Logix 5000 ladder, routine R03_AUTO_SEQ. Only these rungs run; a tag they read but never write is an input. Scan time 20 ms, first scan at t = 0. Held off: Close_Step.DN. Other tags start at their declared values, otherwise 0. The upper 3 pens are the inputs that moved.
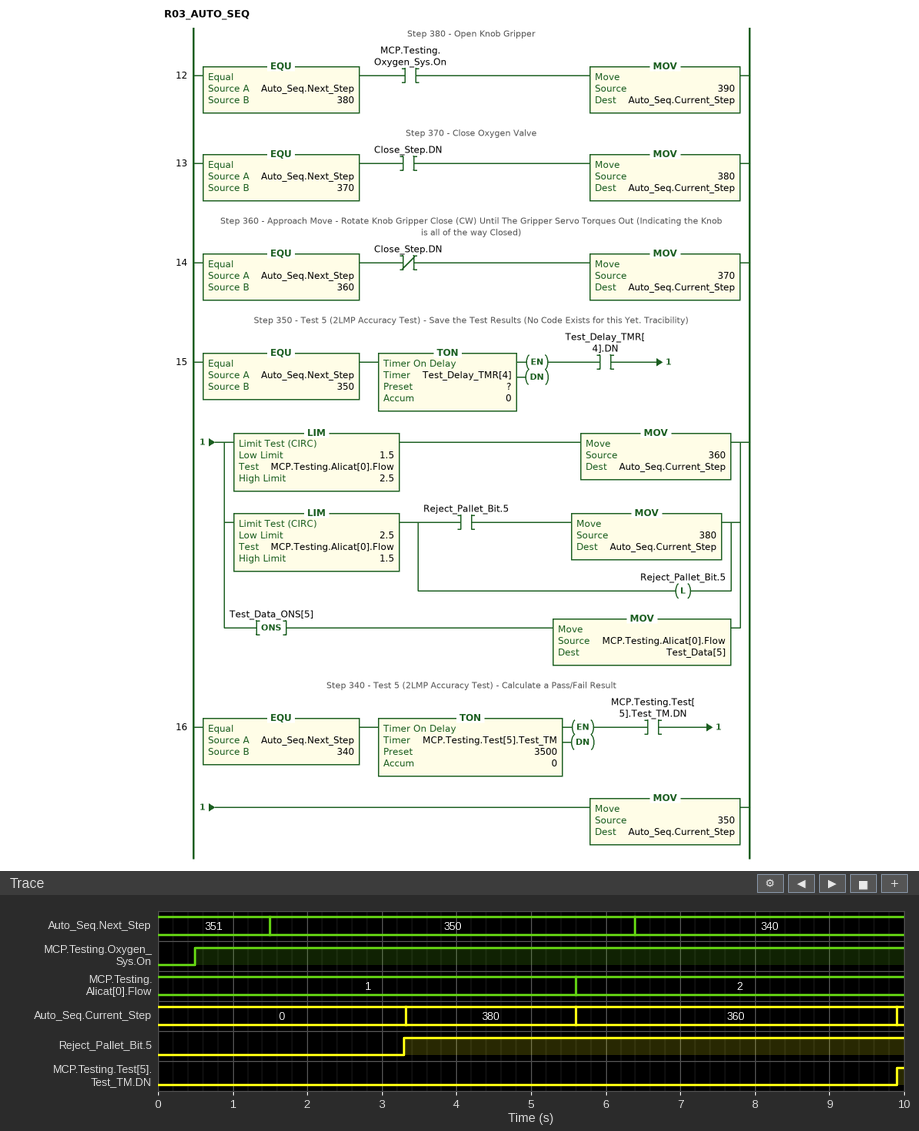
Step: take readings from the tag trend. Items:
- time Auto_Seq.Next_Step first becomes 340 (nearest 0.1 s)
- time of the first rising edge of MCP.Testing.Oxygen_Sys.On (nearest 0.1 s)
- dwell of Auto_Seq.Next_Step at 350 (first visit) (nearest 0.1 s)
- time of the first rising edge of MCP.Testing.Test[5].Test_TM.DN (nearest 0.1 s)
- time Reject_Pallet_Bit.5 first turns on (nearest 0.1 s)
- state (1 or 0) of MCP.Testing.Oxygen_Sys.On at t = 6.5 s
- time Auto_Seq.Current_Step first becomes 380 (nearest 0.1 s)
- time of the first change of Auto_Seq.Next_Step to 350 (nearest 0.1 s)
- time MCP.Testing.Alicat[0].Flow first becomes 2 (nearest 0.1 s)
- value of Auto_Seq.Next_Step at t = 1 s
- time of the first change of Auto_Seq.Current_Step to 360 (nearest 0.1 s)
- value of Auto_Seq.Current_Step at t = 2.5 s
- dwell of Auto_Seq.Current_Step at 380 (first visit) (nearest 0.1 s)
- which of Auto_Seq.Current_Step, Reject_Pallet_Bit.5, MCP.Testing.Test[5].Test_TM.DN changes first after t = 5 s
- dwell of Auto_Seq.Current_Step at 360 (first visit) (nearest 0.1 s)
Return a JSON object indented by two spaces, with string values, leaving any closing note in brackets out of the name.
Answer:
{
  "time Auto_Seq.Next_Step first becomes 340": "6.4 s",
  "time of the first rising edge of MCP.Testing.Oxygen_Sys.On": "0.5 s",
  "dwell of Auto_Seq.Next_Step at 350 (first visit)": "4.9 s",
  "time of the first rising edge of MCP.Testing.Test[5].Test_TM.DN": "9.9 s",
  "time Reject_Pallet_Bit.5 first turns on": "3.3 s",
  "state (1 or 0) of MCP.Testing.Oxygen_Sys.On at t = 6.5 s": "1",
  "time Auto_Seq.Current_Step first becomes 380": "3.3 s",
  "time of the first change of Auto_Seq.Next_Step to 350": "1.5 s",
  "time MCP.Testing.Alicat[0].Flow first becomes 2": "5.6 s",
  "value of Auto_Seq.Next_Step at t = 1 s": "351",
  "time of the first change of Auto_Seq.Current_Step to 360": "5.6 s",
  "value of Auto_Seq.Current_Step at t = 2.5 s": "0",
  "dwell of Auto_Seq.Current_Step at 380 (first visit)": "2.3 s",
  "which of Auto_Seq.Current_Step, Reject_Pallet_Bit.5, MCP.Testing.Test[5].Test_TM.DN changes first after t = 5 s": "Auto_Seq.Current_Step",
  "dwell of Auto_Seq.Current_Step at 360 (first visit)": "4.3 s"
}
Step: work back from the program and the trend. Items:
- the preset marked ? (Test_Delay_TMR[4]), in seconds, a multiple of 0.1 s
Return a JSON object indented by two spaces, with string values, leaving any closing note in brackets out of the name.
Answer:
{
  "the preset marked ? (Test_Delay_TMR[4]), in seconds, a multiple of 0.1 s": "1.8 s"
}
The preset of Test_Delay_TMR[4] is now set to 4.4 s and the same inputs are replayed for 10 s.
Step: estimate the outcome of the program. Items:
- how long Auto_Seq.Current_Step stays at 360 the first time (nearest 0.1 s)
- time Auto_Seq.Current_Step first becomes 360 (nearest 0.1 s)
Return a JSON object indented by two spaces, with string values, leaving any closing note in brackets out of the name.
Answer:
{
  "how long Auto_Seq.Current_Step stays at 360 the first time": "4.0 s",
  "time Auto_Seq.Current_Step first becomes 360": "5.9 s"
}
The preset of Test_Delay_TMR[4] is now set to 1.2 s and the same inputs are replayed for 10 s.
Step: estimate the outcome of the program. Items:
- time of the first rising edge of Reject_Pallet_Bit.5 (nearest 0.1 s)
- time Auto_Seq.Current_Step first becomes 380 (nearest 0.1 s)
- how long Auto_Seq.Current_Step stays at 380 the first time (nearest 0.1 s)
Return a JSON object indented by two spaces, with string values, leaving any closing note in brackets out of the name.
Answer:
{
  "time of the first rising edge of Reject_Pallet_Bit.5": "2.7 s",
  "time Auto_Seq.Current_Step first becomes 380": "2.7 s",
  "how long Auto_Seq.Current_Step stays at 380 the first time": "2.9 s"
}
